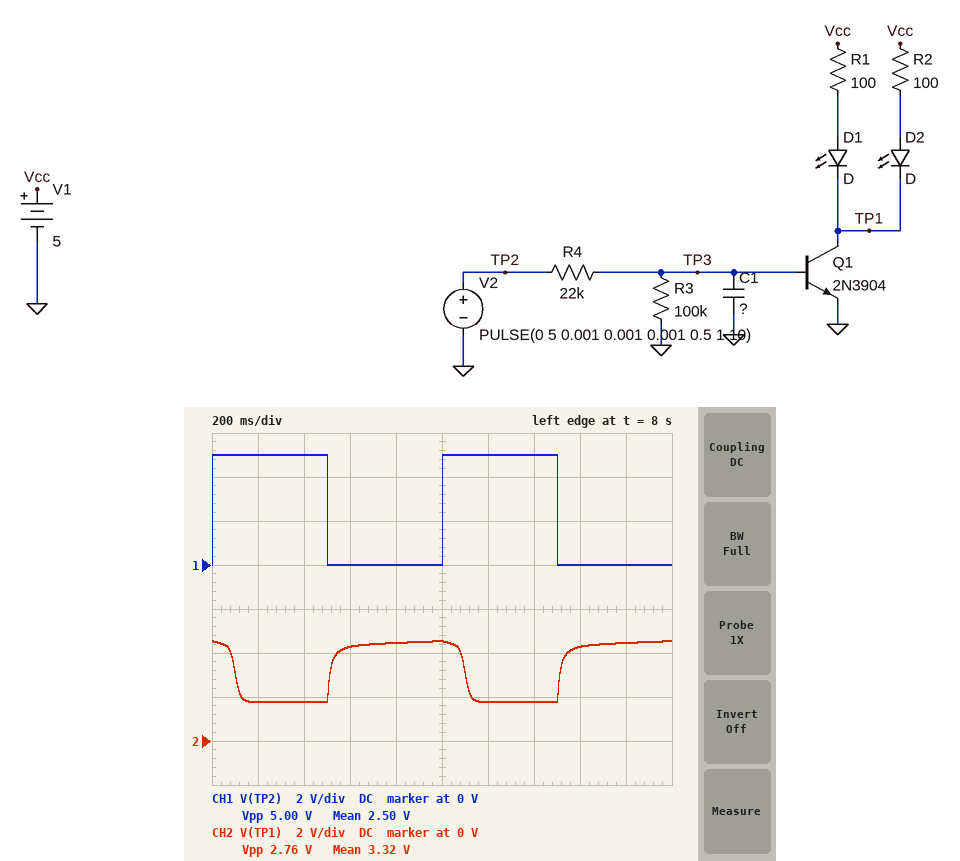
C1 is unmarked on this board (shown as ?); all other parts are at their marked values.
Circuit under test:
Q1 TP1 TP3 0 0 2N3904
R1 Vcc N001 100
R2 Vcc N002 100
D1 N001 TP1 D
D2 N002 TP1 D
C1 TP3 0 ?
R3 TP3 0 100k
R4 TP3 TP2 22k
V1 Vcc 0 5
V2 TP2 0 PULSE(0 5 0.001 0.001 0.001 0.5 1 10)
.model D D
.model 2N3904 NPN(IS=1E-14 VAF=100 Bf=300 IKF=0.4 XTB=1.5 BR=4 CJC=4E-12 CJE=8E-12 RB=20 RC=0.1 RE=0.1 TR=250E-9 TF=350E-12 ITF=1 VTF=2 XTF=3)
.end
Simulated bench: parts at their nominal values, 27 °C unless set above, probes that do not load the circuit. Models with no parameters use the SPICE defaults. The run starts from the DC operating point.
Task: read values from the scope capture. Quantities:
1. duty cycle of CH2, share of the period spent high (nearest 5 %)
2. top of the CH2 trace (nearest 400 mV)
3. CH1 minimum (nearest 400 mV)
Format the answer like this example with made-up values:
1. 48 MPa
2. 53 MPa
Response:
1. 60 %
2. 4.4 V
3. 0 V
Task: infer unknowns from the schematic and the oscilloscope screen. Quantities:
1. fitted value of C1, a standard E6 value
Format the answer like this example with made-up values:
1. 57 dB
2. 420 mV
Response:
1. 68 µF
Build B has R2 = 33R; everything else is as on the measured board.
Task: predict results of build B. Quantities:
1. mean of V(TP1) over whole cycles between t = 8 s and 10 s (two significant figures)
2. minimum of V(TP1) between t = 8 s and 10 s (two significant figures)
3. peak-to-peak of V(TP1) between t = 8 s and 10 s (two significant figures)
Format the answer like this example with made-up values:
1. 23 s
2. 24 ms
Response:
1. 3.8 V
2. 3.0 V
3. 1.5 V
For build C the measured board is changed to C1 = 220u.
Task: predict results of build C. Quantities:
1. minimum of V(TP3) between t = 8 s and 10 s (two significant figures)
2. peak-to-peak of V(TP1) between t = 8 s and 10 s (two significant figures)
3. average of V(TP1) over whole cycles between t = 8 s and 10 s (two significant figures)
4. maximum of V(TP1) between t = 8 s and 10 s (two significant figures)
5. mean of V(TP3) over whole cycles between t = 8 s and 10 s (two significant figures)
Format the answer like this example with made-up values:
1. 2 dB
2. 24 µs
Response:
1. 630 mV
2. 2.6 V
3. 3.3 V
4. 4.4 V
5. 710 mV
